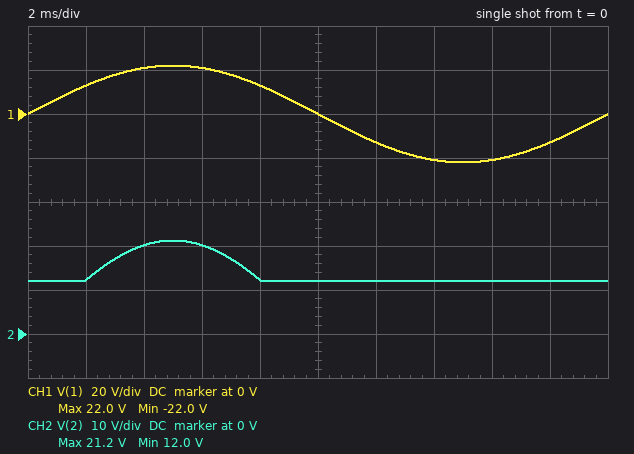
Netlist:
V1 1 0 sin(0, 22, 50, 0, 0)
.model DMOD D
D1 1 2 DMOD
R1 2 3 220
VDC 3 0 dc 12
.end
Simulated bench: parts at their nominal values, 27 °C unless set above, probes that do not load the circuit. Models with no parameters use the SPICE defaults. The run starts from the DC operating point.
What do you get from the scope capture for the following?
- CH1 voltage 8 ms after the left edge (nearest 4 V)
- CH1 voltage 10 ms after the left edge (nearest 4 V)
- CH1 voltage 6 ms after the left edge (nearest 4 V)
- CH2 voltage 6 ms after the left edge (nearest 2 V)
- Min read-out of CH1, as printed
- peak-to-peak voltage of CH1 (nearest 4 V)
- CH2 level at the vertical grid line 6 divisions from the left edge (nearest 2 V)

12 V
0 V
20 V
20 V
-22.0 V
44 V
12 V
